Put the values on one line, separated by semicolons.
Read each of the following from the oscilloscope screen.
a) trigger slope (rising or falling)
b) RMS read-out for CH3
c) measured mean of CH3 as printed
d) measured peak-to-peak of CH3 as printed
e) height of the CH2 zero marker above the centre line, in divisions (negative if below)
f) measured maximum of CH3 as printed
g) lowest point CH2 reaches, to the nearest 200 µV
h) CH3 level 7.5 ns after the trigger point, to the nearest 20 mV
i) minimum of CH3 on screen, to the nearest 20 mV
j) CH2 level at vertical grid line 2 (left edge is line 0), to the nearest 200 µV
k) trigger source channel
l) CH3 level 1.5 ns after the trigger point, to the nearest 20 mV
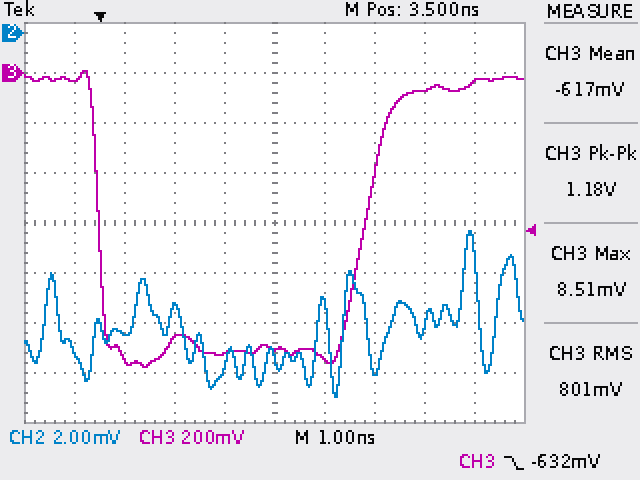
falling; 801 mV; -617 mV; 1.18 V; +3.8 div; 8.51 mV; -14.6 mV; -40 mV; -1.18 V; -12.0 mV; CH3; -1.06 V
